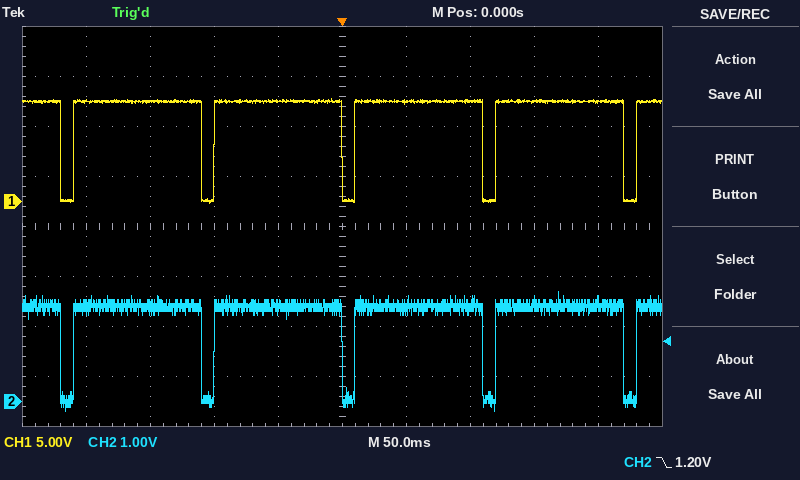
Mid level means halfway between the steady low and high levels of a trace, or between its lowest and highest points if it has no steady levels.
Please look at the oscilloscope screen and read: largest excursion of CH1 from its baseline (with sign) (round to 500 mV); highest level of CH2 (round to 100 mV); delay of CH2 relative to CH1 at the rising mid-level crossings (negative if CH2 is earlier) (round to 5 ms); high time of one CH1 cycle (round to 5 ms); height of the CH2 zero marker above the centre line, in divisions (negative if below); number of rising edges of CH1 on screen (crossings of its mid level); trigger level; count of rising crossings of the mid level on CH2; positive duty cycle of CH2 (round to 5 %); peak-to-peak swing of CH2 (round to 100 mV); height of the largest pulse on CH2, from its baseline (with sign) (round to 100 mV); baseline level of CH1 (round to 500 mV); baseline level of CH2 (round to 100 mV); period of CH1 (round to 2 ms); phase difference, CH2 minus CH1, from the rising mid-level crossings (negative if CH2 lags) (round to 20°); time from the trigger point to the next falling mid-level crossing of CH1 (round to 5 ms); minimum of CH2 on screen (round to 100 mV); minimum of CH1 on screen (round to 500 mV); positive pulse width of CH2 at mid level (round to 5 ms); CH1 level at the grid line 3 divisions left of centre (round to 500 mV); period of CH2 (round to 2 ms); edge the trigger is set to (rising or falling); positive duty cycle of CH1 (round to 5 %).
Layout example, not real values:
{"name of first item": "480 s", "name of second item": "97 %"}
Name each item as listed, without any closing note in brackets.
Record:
{"largest excursion of CH1 from its baseline (with sign)": "-10.0 V", "highest level of CH2": "2.2 V", "delay of CH2 relative to CH1 at the rising mid-level crossings (negative if CH2 is earlier)": "0 ms", "high time of one CH1 cycle": "100 ms", "height of the CH2 zero marker above the centre line, in divisions": "-3.5 div", "number of rising edges of CH1 on screen": "5", "trigger level": "1.20 V", "count of rising crossings of the mid level on CH2": "5", "positive duty cycle of CH2": "90 %", "peak-to-peak swing of CH2": "2.4 V", "height of the largest pulse on CH2, from its baseline (with sign)": "-2.1 V", "baseline level of CH1": "10.0 V", "baseline level of CH2": "1.9 V", "period of CH1": "110 ms", "phase difference, CH2 minus CH1, from the rising mid-level crossings (negative if CH2 lags)": "0°", "time from the trigger point to the next falling mid-level crossing of CH1": "110 ms", "minimum of CH2 on screen": "-200 mV", "minimum of CH1 on screen": "0.0 V", "positive pulse width of CH2 at mid level": "100 ms", "CH1 level at the grid line 3 divisions left of centre": "10.0 V", "period of CH2": "110 ms", "edge the trigger is set to": "falling", "positive duty cycle of CH1": "90 %"}
